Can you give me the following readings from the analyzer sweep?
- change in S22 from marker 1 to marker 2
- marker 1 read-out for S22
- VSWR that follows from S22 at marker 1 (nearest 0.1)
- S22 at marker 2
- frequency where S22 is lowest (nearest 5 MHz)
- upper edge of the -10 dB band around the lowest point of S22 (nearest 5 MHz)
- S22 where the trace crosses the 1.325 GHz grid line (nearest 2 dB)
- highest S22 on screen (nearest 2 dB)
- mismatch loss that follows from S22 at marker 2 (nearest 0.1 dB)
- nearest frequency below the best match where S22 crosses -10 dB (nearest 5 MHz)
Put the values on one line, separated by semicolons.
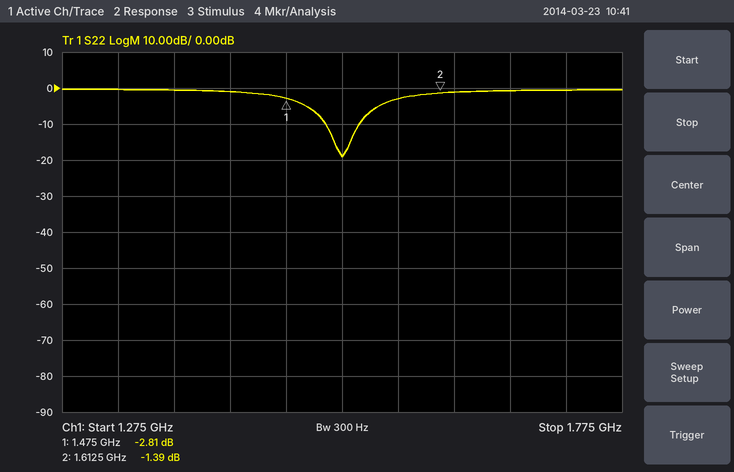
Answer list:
1.42 dB; -2.81 dB; 6.2; -1.39 dB; 1.525 GHz; 1.540 GHz; 0 dB; 0 dB; 5.6 dB; 1.510 GHz
